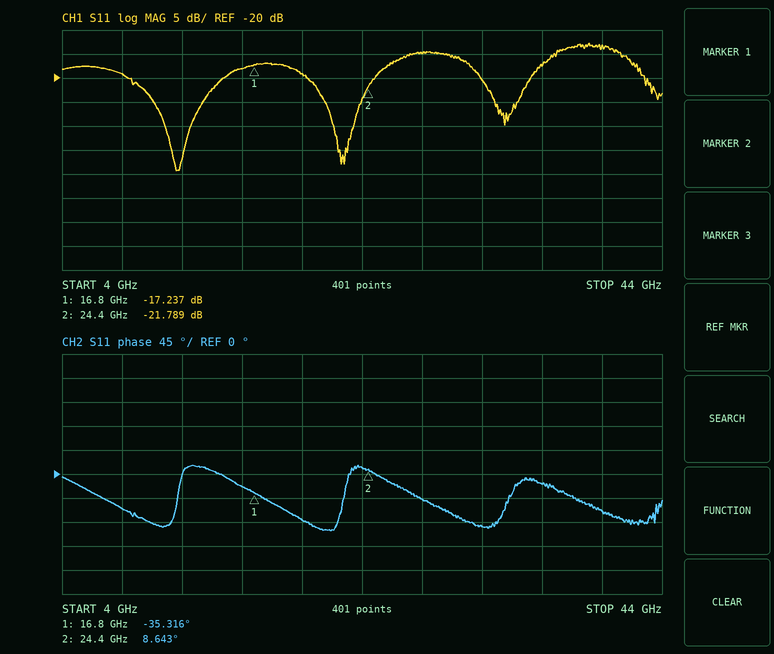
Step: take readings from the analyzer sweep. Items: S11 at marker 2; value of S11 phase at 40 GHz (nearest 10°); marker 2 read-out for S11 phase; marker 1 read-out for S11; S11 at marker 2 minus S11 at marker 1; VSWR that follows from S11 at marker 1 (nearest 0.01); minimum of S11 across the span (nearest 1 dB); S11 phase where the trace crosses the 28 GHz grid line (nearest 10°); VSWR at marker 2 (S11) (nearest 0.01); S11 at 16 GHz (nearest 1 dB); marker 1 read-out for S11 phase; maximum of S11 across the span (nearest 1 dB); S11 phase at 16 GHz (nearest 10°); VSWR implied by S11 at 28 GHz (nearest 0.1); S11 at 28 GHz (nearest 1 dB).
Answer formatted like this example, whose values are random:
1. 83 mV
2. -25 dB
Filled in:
1. -21.789 dB
2. -70°
3. 8.643°
4. -17.237 dB
5. -4.552 dB
6. 1.32
7. -39 dB
8. -50°
9. 1.18
10. -18 dB
11. -35.316°
12. -13 dB
13. -20°
14. 1.4
15. -15 dB
